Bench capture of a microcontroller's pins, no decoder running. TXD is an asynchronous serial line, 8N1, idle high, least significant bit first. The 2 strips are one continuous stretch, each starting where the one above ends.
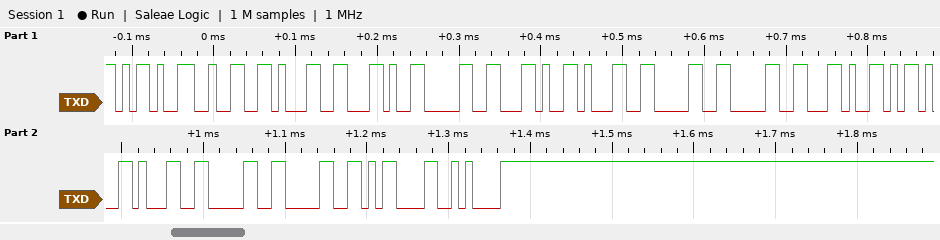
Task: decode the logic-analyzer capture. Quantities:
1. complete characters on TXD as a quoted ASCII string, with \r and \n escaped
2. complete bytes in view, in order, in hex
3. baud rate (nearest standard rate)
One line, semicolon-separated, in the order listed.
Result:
"-21,0,100,-100\r\n"; 2D 32 31 2C 30 2C 31 30 30 2C 2D 31 30 30 0D 0A; 115200 baud
